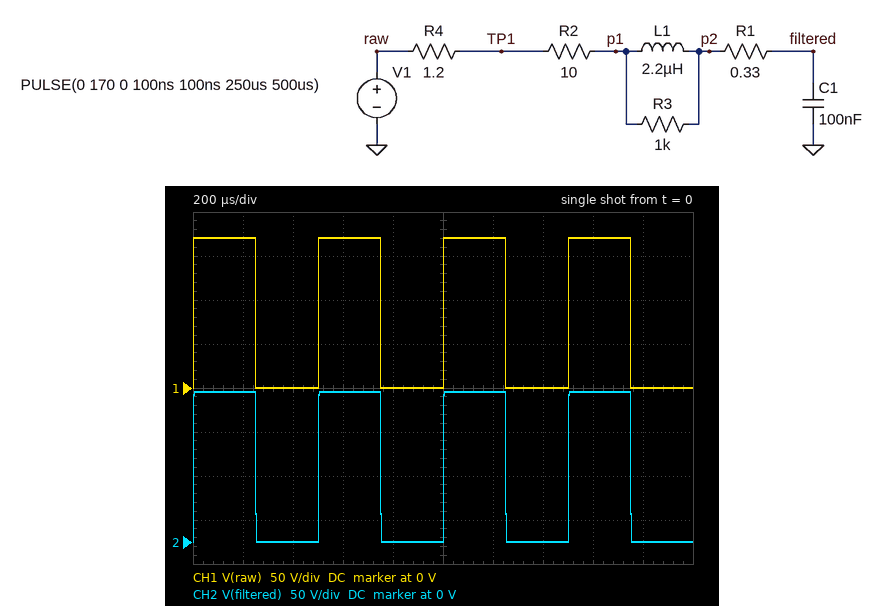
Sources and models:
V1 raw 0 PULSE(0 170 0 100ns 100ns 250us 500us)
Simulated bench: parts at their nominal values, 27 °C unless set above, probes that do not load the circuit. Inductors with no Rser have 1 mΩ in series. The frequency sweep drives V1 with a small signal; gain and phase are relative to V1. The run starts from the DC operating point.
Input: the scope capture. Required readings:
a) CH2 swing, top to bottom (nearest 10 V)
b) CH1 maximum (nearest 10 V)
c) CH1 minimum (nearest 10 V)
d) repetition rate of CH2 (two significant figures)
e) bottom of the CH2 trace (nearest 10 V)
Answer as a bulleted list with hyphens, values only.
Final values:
- 170 V
- 170 V
- 0 V
- 2.0 kHz
- 0 V
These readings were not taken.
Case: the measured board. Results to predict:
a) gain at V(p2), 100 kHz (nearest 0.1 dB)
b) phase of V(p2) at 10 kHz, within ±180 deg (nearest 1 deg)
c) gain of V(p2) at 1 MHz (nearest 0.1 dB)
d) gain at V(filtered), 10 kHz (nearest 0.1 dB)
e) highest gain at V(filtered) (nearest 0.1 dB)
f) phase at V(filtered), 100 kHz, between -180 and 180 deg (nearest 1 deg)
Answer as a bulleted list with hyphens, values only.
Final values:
- -1.3 dB
- -4 deg
- -20.4 dB
- 0 dB
- 0 dB
- -38 deg
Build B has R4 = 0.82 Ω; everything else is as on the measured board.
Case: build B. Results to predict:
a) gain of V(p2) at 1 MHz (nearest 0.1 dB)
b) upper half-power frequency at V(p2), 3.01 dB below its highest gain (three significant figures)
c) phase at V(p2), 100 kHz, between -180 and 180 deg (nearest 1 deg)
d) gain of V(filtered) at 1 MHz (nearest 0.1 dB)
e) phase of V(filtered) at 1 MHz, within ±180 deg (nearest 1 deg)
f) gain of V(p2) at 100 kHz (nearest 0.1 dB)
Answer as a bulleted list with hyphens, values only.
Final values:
- -20.2 dB
- 172 kHz
- -36 deg
- -20.4 dB
- -137 deg
- -1.2 dB
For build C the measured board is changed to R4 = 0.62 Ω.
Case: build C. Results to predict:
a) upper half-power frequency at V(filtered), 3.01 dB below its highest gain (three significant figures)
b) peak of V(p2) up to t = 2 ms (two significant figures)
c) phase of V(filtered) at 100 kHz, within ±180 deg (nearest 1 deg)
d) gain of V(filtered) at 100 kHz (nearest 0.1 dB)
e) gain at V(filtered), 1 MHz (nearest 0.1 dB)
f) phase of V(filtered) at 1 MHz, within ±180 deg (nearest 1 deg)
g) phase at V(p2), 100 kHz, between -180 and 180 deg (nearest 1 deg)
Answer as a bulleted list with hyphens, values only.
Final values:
- 176 kHz
- 170 V
- -37 deg
- -1.2 dB
- -20.3 dB
- -138 deg
- -36 deg
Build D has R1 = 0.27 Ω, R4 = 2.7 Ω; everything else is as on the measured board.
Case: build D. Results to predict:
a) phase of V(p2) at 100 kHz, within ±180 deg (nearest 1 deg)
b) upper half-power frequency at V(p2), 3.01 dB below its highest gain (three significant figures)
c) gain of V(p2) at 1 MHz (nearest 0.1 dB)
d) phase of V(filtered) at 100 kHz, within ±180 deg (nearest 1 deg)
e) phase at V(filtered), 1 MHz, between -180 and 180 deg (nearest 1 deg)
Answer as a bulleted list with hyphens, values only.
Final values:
- -41 deg
- 141 kHz
- -20.9 dB
- -42 deg
- -133 deg
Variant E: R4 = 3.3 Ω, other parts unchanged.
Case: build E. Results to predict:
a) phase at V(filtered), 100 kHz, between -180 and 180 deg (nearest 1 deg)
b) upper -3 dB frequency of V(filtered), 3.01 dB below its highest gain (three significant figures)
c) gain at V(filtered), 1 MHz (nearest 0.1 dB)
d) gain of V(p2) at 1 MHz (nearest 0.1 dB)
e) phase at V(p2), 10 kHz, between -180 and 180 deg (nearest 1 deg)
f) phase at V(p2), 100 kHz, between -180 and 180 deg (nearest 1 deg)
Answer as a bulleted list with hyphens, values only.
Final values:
- -43 deg
- 132 kHz
- -21.3 dB
- -21.1 dB
- -5 deg
- -42 deg
